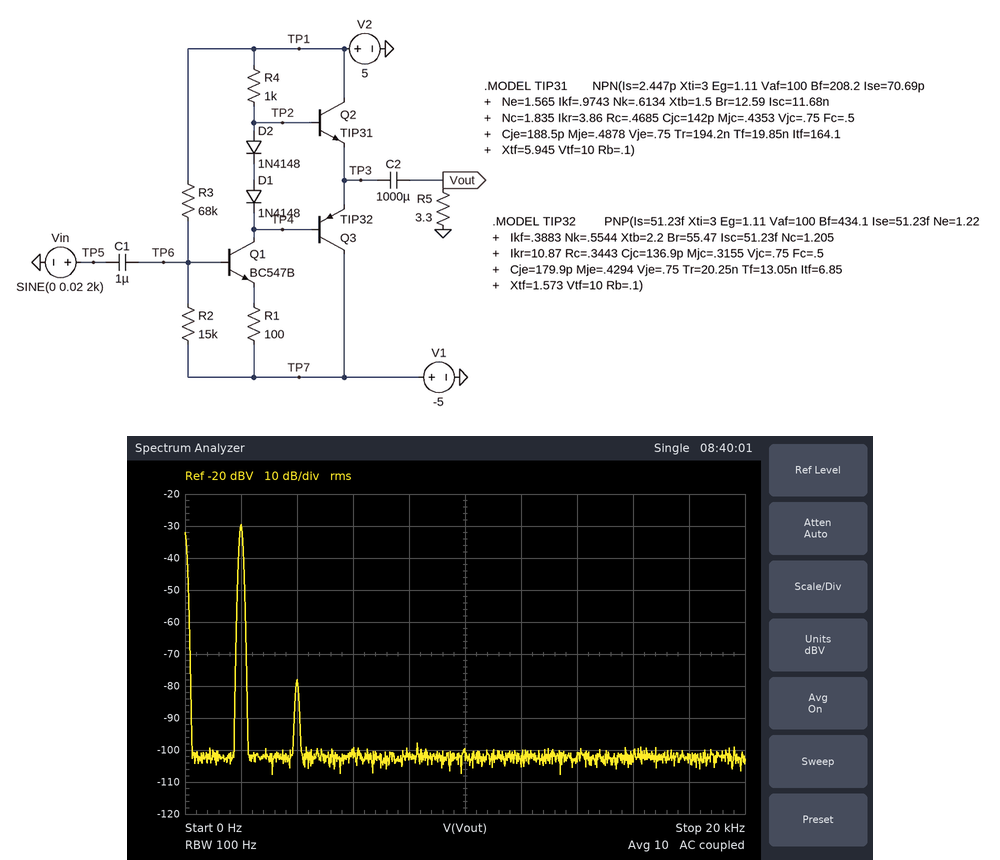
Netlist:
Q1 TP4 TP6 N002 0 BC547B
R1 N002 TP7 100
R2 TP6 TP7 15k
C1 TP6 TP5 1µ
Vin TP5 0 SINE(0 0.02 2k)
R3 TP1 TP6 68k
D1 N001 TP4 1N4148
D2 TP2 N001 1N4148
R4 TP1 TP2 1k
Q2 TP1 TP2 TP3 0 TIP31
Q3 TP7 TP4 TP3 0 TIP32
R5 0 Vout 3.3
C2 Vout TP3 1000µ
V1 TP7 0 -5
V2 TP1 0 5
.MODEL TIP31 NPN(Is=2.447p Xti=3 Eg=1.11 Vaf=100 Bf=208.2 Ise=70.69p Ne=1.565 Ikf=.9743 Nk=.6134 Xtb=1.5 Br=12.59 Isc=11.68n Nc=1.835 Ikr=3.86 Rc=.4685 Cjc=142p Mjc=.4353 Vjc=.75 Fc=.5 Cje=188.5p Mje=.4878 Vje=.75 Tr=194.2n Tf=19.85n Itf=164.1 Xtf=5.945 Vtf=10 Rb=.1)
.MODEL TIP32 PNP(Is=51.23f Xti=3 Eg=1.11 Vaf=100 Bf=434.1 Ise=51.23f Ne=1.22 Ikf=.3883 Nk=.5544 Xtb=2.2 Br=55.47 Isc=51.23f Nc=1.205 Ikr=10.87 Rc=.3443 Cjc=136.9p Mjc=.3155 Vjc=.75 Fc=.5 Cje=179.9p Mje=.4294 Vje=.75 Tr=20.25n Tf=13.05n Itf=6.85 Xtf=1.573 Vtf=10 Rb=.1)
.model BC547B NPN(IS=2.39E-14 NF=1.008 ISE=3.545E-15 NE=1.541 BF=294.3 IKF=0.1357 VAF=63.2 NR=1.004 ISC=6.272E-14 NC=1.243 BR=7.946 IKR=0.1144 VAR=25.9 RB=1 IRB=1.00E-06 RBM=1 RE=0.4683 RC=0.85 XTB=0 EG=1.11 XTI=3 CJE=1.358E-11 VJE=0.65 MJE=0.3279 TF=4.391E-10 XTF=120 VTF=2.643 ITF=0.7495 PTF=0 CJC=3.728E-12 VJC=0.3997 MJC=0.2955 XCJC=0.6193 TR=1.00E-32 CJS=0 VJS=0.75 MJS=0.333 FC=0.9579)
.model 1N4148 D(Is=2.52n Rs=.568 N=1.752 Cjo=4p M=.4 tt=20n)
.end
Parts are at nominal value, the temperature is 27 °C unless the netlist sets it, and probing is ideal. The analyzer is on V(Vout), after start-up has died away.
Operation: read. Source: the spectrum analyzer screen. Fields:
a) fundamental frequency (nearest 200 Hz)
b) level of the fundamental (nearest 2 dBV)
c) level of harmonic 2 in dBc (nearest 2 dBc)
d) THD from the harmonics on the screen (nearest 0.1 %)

2.0 kHz
-30 dBV
-48 dBc
0.4 %
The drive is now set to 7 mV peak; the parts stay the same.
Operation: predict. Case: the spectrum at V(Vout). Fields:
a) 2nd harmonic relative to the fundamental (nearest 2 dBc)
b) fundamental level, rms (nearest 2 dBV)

-58 dBc
-38 dBV
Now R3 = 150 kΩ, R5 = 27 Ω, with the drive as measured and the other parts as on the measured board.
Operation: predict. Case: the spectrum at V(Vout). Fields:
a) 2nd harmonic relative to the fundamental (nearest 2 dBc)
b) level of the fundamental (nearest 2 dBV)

-40 dBc
-22 dBV
